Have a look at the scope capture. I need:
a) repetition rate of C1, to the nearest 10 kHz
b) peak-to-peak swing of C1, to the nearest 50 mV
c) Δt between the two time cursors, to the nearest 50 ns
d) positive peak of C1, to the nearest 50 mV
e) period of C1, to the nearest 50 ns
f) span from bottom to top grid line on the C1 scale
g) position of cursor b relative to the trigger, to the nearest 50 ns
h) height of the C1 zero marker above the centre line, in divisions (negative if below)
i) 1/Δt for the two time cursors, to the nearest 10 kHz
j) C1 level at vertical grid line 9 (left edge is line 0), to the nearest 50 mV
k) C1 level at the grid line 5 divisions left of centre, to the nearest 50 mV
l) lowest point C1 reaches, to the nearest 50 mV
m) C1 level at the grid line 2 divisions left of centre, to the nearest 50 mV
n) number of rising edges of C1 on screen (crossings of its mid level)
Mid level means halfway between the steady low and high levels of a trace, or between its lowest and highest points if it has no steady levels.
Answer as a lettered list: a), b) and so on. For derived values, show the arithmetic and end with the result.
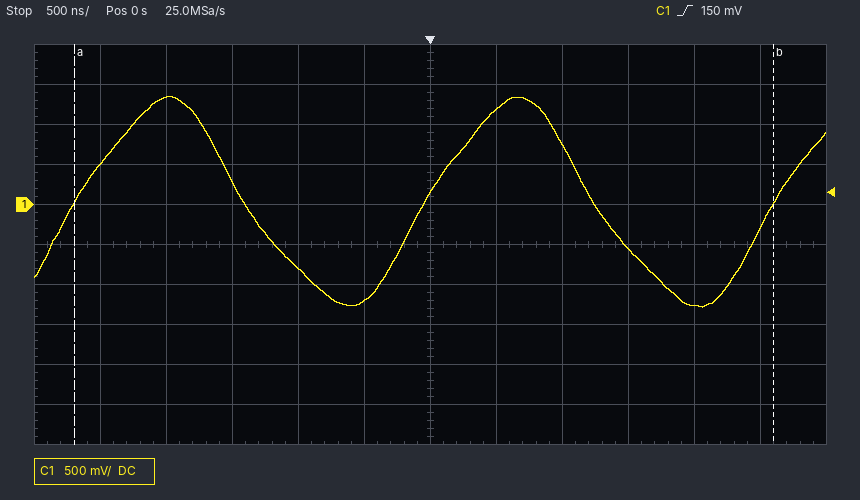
a) 1 / 2.65 µs ≈ 377 kHz, so 380 kHz to the nearest 10 kHz
b) 1.35 V − (-1.30 V) = 2.65 V
c) 5.30 µs
d) 1.35 V
e) 2.65 µs
f) 5 V
g) +2.60 µs
h) +1.0 div
i) 1 / 5.30 µs ≈ 190 kHz
j) -550 mV
k) 500 mV
l) -1.30 V
m) -800 mV
n) 3
